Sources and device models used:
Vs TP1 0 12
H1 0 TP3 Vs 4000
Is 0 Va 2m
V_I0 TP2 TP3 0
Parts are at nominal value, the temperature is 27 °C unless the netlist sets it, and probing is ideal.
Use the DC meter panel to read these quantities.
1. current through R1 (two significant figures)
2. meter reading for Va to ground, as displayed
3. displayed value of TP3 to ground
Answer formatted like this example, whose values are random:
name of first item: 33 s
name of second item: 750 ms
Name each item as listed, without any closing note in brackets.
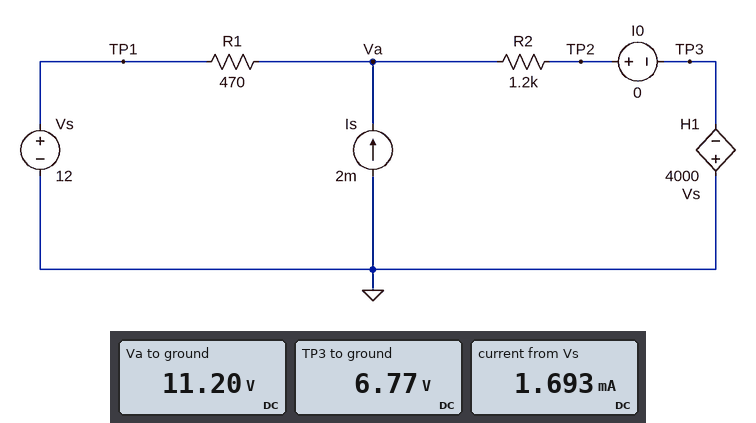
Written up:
current through R1: 1.7 mA
meter reading for Va to ground, as displayed: 11.20 V
displayed value of TP3 to ground: 6.77 V
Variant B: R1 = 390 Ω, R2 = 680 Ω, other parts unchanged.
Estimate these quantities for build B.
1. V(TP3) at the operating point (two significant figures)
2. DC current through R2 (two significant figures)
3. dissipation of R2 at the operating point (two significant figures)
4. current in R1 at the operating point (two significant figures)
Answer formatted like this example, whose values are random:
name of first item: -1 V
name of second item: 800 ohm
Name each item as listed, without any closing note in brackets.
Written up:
V(TP3) at the operating point: 8.4 V
DC current through R2: 4.1 mA
dissipation of R2 at the operating point: 11 mW
current in R1 at the operating point: 2.1 mA
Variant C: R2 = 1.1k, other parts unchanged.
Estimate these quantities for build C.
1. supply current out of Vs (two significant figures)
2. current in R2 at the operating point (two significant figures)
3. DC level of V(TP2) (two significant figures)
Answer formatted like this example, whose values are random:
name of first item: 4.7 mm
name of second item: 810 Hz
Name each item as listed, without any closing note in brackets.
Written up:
supply current out of Vs: 1.8 mA
current in R2 at the operating point: 3.8 mA
DC level of V(TP2): 7.0 V
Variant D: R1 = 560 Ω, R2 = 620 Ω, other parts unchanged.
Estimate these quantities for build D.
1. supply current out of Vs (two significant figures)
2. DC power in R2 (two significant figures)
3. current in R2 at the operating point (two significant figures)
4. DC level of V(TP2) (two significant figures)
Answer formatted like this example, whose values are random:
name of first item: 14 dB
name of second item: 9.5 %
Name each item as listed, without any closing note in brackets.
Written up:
supply current out of Vs: 2.1 mA
DC power in R2: 10 mW
current in R2 at the operating point: 4.1 mA
DC level of V(TP2): 8.3 V
